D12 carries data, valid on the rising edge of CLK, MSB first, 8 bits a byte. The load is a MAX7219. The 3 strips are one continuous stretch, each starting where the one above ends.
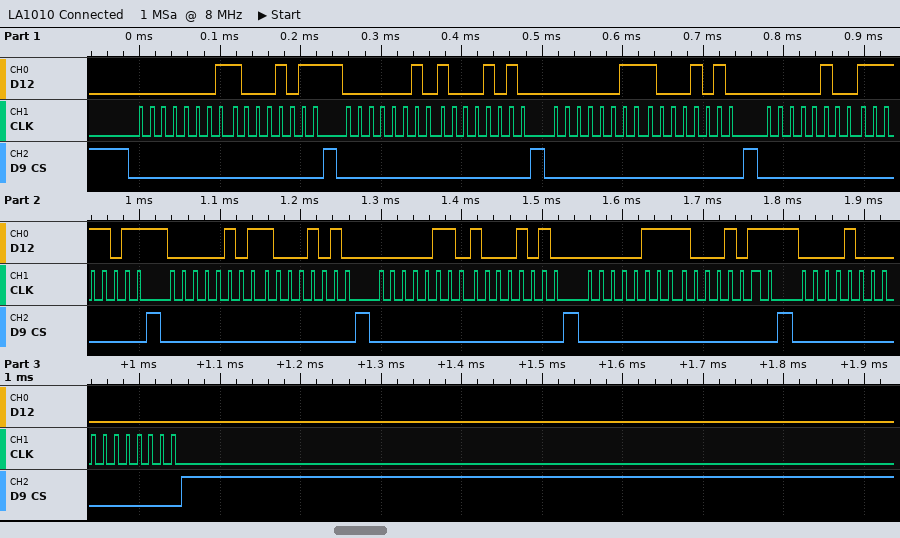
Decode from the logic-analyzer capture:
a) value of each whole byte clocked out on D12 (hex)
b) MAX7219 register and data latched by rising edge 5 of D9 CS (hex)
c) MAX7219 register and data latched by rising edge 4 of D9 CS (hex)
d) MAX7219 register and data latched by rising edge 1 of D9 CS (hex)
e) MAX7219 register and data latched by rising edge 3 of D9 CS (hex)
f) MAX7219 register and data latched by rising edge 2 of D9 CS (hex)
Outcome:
0x01 0x8B 0x02 0x8A 0x03 0x8A 0x04 0xFB 0x05 0x8A 0x06 0x8A 0x07 0x8B 0x08 0x00
register 0x5, data 0x8A
register 0x4, data 0xFB
register 0x1, data 0x8B
register 0x3, data 0x8A
register 0x2, data 0x8A
